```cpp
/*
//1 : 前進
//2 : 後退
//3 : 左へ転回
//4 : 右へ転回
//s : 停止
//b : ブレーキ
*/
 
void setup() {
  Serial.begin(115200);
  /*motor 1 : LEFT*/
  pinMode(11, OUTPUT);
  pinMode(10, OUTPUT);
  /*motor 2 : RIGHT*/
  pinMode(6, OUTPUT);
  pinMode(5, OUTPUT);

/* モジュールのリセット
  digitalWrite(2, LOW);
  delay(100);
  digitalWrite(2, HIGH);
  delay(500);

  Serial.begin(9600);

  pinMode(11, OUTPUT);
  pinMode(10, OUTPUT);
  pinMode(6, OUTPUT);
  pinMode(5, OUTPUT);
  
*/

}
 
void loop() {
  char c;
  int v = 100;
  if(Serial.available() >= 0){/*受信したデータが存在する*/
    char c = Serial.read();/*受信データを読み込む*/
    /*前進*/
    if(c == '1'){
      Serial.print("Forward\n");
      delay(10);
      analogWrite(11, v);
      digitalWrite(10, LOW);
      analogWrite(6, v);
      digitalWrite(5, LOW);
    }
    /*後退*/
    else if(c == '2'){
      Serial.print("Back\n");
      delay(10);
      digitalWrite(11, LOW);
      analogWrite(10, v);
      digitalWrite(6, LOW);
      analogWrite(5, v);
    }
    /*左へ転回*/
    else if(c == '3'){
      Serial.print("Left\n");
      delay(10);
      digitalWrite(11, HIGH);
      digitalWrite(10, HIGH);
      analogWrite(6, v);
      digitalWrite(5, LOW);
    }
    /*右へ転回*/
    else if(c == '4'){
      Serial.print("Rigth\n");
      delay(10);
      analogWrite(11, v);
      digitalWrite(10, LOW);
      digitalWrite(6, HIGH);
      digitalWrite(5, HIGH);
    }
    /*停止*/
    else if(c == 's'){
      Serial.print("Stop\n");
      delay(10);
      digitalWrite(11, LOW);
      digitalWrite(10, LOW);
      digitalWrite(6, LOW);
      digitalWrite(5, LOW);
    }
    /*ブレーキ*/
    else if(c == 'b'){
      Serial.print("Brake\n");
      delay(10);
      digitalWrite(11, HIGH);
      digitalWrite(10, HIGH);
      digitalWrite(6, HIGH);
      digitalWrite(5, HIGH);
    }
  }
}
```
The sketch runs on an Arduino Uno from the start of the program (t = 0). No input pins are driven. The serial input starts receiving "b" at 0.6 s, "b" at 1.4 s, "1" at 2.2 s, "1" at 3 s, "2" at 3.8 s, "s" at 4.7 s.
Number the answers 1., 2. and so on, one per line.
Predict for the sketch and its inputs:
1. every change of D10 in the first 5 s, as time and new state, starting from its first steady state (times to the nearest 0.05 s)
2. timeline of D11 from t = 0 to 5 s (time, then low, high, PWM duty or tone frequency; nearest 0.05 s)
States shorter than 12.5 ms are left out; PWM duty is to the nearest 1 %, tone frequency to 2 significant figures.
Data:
1. 0 s low; 0.6 s high; 2.2 s low; 3.8 s PWM 39 %; 4.7 s low
2. 0 s low; 0.6 s high; 2.2 s PWM 39 %; 3.8 s low
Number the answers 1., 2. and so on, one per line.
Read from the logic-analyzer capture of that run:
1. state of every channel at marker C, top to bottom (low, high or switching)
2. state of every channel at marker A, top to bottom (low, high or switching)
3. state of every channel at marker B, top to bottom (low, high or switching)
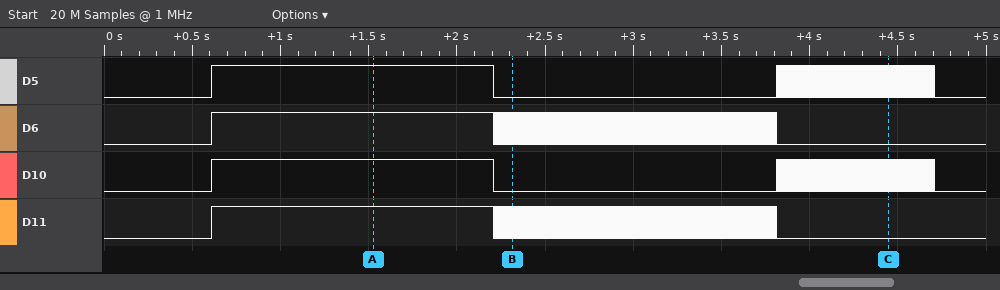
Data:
1. D5 switching, D6 low, D10 switching, D11 low
2. D5 high, D6 high, D10 high, D11 high
3. D5 low, D6 switching, D10 low, D11 switching
